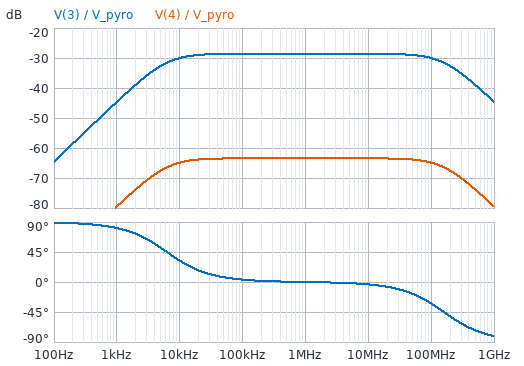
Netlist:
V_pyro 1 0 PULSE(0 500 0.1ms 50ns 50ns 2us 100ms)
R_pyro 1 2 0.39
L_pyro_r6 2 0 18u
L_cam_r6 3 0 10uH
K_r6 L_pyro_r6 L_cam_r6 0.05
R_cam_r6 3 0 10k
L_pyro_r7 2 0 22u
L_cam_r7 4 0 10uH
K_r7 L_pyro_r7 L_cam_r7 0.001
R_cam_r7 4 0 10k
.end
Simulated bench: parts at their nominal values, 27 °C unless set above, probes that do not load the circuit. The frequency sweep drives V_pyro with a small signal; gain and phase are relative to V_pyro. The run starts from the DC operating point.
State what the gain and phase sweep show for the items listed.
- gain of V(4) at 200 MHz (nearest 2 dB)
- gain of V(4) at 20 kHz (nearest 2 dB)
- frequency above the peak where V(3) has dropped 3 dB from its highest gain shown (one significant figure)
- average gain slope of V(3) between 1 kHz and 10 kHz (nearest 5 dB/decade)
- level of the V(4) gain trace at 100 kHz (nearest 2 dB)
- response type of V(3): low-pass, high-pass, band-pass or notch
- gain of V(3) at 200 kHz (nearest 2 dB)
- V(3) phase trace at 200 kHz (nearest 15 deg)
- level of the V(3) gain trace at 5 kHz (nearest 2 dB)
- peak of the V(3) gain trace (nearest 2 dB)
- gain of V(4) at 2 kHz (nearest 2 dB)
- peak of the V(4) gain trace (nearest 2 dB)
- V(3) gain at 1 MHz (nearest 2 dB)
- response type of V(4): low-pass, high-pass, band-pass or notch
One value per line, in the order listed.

-68 dB
-64 dB
200 MHz
15 dB/decade
-64 dB
band-pass
-28 dB
0 deg
-32 dB
-28 dB
-74 dB
-64 dB
-28 dB
band-pass
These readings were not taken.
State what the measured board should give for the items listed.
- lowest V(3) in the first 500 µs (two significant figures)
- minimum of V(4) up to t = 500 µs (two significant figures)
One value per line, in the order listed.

-1.5 V
-27 mV
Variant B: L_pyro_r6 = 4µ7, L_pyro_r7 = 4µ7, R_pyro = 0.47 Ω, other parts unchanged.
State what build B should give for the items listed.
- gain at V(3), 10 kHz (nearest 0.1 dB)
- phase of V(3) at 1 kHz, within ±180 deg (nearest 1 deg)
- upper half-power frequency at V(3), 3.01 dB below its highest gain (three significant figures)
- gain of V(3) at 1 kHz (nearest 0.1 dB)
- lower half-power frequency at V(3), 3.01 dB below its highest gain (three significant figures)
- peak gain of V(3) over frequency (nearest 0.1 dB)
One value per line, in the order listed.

-33.2 dB
88 deg
160 MHz
-52.8 dB
31.8 kHz
-22.7 dB
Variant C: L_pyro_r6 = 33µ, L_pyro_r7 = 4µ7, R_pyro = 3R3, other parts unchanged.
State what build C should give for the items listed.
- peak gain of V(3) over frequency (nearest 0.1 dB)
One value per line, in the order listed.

-31.2 dB
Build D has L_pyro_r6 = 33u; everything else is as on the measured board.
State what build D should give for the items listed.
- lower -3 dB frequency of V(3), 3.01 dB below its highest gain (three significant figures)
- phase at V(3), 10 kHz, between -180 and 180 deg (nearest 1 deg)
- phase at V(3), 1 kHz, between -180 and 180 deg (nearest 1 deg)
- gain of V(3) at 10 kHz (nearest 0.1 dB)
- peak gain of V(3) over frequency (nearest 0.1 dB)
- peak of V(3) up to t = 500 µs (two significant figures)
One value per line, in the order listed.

4.70 kHz
25 deg
78 deg
-32.1 dB
-31.2 dB
14 V
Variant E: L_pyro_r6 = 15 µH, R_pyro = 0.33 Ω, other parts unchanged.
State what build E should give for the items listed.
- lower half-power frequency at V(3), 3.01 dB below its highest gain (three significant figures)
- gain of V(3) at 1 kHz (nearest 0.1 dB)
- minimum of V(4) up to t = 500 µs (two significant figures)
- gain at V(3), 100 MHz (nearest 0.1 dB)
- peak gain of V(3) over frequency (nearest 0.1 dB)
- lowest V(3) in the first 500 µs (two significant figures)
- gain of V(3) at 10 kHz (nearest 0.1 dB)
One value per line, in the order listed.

5.89 kHz
-43.3 dB
-25 mV
-29.2 dB
-27.8 dB
-1.5 V
-29.1 dB
